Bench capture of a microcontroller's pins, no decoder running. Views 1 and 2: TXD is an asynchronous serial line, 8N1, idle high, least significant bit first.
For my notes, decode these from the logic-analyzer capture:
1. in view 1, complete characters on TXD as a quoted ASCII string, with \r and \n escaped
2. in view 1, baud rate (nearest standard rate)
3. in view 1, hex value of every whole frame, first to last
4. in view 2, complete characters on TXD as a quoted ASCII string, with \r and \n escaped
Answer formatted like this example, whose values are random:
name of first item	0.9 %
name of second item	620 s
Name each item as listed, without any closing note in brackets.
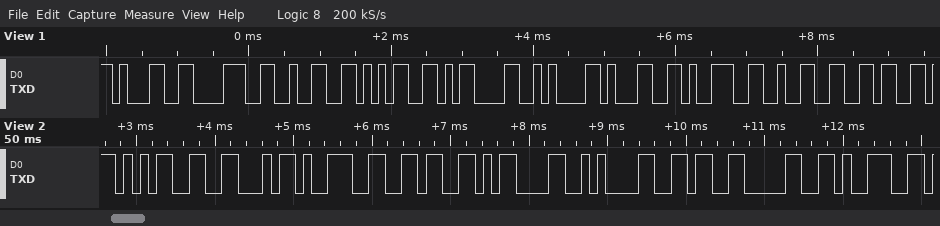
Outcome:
in view 1, complete characters on TXD as a quoted ASCII string, with \r and \n escaped	"1825\r\n1926"
in view 1, baud rate	9600 baud
in view 1, hex value of every whole frame, first to last	31 38 32 35 0D 0A 31 39 32 36
in view 2, complete characters on TXD as a quoted ASCII string, with \r and \n escaped	"5F96\r\n609"
